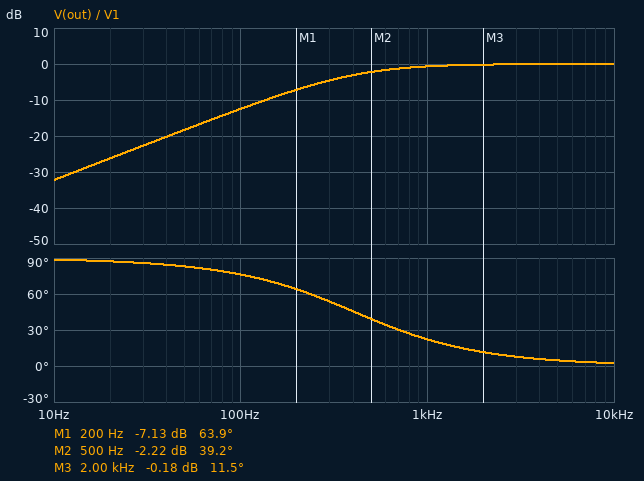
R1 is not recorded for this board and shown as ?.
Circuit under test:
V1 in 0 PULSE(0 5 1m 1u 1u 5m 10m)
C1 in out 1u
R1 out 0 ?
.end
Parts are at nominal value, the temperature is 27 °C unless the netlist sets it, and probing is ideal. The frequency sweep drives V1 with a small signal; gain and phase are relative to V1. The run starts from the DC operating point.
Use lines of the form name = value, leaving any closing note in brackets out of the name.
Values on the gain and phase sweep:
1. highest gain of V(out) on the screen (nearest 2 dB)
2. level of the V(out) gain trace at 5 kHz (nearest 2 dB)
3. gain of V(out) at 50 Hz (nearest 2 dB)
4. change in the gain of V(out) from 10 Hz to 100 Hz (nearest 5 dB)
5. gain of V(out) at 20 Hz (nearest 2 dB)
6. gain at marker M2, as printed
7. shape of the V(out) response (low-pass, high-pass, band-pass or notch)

highest gain of V(out) on the screen = 0 dB
level of the V(out) gain trace at 5 kHz = 0 dB
gain of V(out) at 50 Hz = -18 dB
change in the gain of V(out) from 10 Hz to 100 Hz = 20 dB
gain of V(out) at 20 Hz = -26 dB
gain at marker M2, as printed = -2.22 dB
shape of the V(out) response = high-pass
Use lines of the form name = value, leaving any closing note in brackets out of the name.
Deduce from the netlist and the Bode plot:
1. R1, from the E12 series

R1, from the E12 series = 390 Ω
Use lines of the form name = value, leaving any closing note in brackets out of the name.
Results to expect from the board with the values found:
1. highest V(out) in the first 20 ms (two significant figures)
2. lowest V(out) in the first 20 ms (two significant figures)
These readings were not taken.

highest V(out) in the first 20 ms = 5.0 V
lowest V(out) in the first 20 ms = -5.0 V
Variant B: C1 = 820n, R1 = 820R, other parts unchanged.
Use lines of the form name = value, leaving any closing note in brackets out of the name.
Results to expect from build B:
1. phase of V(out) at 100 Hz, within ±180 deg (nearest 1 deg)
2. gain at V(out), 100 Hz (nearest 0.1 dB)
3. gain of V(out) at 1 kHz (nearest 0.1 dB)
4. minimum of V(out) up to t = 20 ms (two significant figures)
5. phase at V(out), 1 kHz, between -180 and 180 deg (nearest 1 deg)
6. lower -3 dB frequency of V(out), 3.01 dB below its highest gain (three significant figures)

phase of V(out) at 100 Hz, within ±180 deg = 67 deg
gain at V(out), 100 Hz = -8.2 dB
gain of V(out) at 1 kHz = -0.2 dB
minimum of V(out) up to t = 20 ms = -5.0 V
phase at V(out), 1 kHz, between -180 and 180 deg = 13 deg
lower -3 dB frequency of V(out), 3.01 dB below its highest gain = 237 Hz
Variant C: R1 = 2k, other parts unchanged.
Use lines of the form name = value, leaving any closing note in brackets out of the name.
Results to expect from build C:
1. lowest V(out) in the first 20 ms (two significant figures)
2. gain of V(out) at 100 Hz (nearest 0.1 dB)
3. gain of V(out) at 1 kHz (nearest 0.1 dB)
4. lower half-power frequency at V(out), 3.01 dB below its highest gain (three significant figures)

lowest V(out) in the first 20 ms = -4.6 V
gain of V(out) at 100 Hz = -2.1 dB
gain of V(out) at 1 kHz = 0 dB
lower half-power frequency at V(out), 3.01 dB below its highest gain = 79.6 Hz
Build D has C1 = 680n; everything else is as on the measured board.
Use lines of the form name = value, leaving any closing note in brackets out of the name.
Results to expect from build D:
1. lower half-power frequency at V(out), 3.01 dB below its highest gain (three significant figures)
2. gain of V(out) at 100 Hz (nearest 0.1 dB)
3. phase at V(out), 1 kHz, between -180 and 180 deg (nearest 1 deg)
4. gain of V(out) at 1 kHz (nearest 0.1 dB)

lower half-power frequency at V(out), 3.01 dB below its highest gain = 600 Hz
gain of V(out) at 100 Hz = -15.7 dB
phase at V(out), 1 kHz, between -180 and 180 deg = 31 deg
gain of V(out) at 1 kHz = -1.3 dB
